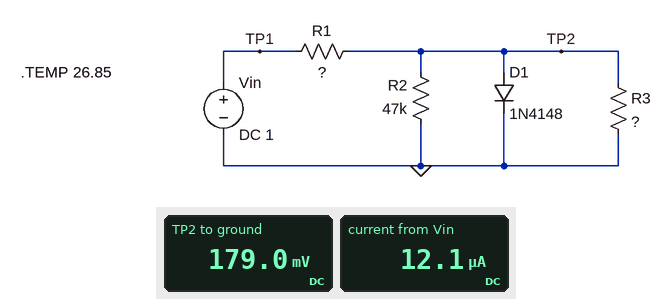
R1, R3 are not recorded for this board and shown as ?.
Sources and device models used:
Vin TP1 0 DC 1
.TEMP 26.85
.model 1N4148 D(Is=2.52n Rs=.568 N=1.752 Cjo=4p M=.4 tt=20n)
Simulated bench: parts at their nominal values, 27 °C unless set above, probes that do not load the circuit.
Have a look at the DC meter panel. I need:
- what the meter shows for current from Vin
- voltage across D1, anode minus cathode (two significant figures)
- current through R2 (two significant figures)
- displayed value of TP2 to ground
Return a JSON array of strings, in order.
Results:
["12.1 µA", "180 mV", "3.8 µA", "179.0 mV"]
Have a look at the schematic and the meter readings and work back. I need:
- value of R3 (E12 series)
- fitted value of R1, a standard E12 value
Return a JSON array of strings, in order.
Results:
["22 kΩ", "68 kΩ"]
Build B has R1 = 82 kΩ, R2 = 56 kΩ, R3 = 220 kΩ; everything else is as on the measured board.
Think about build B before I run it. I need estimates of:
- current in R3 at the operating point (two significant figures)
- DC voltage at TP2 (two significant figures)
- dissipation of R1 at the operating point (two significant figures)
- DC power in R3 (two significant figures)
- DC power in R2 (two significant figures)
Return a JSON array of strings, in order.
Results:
["1.4 µA", "300 mV", "6.0 µW", "410 nW", "1.6 µW"]
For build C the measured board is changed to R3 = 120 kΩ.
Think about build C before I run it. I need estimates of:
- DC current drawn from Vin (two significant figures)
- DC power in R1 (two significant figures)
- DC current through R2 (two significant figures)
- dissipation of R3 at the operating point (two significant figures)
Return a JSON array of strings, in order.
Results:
["10 µA", "7.3 µW", "6.3 µA", "720 nW"]
